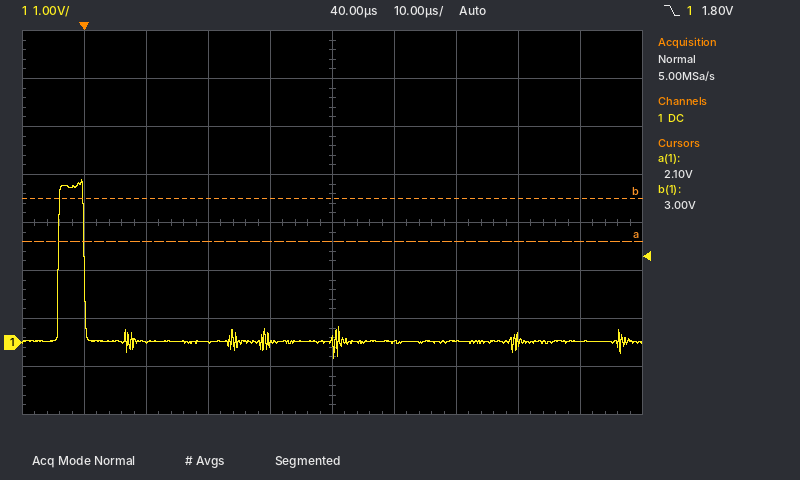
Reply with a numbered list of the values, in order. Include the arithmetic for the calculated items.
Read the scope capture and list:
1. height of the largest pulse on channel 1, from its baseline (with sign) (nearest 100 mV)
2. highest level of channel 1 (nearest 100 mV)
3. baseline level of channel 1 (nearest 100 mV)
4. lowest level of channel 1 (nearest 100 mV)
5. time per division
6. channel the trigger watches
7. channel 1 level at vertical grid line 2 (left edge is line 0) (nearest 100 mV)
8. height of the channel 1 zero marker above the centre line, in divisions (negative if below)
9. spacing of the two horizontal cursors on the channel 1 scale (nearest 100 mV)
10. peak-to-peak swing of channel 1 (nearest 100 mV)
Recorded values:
1. 3.4 V − (0.0 V) = +3.4 V
2. 3.4 V
3. 0.0 V
4. -300 mV
5. 10 µs
6. channel 1
7. 0.0 V
8. -2.5 div
9. 900 mV
10. 3.4 V − (-300 mV) = 3.7 V
